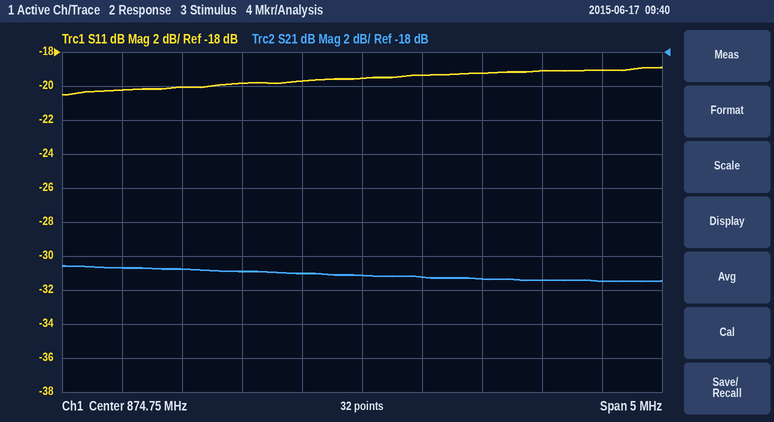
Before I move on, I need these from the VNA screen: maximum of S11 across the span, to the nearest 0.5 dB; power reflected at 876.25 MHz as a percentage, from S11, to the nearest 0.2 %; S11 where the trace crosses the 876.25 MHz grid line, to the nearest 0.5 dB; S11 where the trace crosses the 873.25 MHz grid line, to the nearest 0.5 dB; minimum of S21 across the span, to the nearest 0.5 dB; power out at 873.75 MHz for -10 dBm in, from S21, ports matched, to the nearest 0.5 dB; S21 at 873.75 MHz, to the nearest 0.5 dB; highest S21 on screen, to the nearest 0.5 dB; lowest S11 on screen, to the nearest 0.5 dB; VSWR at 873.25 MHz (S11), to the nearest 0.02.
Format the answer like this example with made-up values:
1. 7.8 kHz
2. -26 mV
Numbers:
1. -19.0 dB
2. 1.2 %
3. -19.0 dB
4. -20.0 dB
5. -31.5 dB
6. -41.0 dBm
7. -31.0 dB
8. -30.5 dB
9. -20.5 dB
10. 1.22
